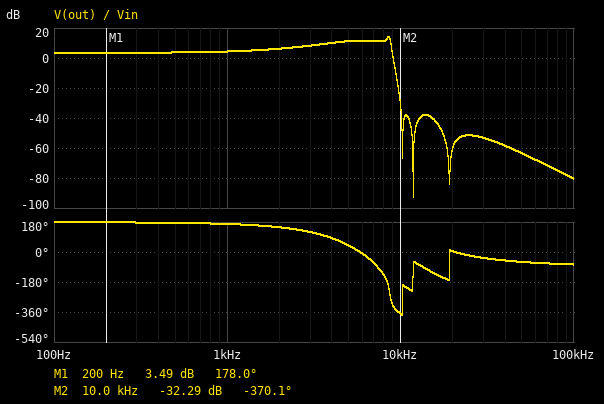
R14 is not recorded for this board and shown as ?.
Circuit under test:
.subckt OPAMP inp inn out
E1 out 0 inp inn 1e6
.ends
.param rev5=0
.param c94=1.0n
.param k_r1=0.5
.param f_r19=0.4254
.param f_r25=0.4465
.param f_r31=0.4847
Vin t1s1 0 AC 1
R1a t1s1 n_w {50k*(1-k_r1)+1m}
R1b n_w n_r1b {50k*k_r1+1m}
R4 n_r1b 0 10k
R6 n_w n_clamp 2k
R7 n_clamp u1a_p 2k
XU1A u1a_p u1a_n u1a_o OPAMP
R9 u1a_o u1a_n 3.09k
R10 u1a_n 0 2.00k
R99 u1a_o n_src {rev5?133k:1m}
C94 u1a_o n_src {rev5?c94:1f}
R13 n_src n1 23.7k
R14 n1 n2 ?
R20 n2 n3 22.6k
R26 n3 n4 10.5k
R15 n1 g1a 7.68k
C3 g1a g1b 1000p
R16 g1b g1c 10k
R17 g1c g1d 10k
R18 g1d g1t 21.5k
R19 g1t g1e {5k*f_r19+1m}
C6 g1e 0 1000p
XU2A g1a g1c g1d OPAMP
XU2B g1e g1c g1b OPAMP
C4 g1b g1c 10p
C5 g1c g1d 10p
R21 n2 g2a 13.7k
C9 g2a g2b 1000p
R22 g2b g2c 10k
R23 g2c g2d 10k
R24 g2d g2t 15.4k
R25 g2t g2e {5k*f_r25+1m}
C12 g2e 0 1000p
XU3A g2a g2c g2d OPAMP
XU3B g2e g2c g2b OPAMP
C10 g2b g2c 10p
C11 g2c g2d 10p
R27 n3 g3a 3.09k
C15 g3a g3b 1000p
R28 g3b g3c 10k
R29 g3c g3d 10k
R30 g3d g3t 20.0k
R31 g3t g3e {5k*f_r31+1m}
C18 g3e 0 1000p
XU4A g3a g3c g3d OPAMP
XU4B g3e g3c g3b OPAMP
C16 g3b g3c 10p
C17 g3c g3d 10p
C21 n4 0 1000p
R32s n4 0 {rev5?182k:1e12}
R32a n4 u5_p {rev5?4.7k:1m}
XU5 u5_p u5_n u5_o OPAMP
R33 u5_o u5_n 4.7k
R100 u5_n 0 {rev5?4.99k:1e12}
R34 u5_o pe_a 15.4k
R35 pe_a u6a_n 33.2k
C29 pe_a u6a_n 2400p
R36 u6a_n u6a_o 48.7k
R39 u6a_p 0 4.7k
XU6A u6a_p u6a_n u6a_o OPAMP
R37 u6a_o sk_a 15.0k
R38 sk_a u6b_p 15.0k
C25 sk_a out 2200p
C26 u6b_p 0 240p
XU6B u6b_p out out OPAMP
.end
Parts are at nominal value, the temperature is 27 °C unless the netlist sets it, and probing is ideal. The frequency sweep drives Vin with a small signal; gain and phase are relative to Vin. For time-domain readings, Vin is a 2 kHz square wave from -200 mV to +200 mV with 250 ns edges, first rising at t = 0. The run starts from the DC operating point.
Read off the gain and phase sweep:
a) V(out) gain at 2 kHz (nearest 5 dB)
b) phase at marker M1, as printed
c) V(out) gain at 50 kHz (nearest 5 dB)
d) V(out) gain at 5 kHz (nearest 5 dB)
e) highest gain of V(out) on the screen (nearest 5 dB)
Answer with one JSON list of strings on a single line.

["5 dB", "178.0 deg", "-65 dB", "10 dB", "15 dB"]
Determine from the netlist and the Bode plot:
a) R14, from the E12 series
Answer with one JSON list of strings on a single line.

["18 kΩ"]
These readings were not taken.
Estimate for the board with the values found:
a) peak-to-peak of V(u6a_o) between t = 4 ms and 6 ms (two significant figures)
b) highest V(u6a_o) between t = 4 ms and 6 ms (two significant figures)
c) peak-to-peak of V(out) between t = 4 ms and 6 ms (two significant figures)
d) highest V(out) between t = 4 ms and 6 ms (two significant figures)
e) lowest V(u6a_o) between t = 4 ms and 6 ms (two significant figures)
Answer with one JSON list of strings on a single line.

["1.5 V", "740 mV", "1.6 V", "790 mV", "-740 mV"]
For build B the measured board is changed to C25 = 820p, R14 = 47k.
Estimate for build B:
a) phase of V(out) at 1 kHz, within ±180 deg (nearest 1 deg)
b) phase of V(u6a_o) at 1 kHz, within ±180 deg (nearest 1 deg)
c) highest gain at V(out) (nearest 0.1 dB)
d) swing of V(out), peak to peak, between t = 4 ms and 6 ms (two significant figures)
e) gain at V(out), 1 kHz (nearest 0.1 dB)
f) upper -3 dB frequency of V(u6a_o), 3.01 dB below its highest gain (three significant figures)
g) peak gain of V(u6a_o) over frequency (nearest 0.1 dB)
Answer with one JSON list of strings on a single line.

["159 deg", "161 deg", "18.1 dB", "1.3 V", "3.9 dB", "7.14 kHz", "17.8 dB"]
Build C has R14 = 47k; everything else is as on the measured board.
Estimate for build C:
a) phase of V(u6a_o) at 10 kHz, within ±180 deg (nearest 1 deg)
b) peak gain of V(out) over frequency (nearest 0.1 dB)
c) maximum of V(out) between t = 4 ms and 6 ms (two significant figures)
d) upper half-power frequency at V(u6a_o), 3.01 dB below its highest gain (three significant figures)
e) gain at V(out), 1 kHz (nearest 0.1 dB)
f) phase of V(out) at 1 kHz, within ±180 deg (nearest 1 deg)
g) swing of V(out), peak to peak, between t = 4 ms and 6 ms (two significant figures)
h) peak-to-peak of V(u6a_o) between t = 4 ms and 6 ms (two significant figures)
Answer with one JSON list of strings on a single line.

["30 deg", "19.3 dB", "690 mV", "7.14 kHz", "3.9 dB", "159 deg", "1.4 V", "1.3 V"]
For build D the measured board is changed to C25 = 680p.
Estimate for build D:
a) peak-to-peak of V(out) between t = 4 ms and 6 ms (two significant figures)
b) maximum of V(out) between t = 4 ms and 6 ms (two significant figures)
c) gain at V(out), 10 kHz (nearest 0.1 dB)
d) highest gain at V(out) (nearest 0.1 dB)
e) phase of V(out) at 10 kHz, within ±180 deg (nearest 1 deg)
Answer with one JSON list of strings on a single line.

["1.5 V", "740 mV", "-35.1 dB", "12.2 dB", "2 deg"]
